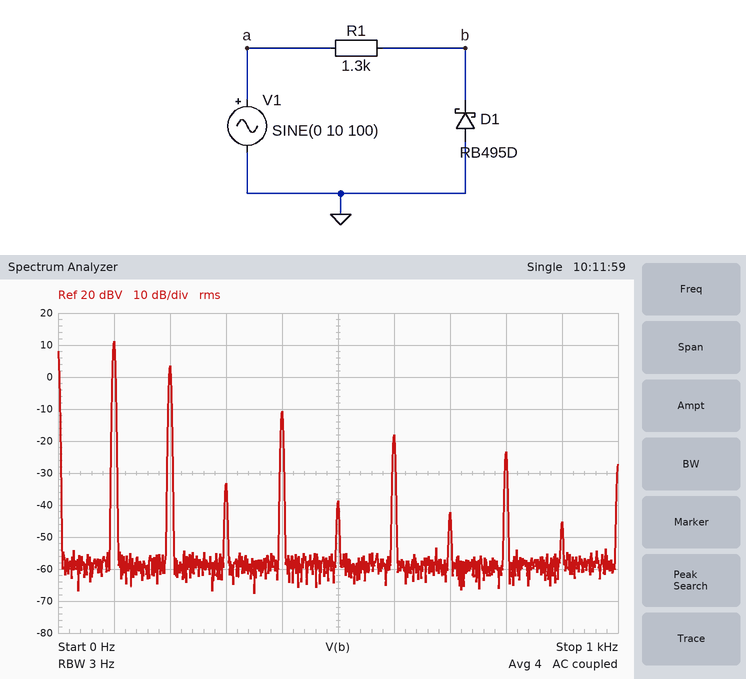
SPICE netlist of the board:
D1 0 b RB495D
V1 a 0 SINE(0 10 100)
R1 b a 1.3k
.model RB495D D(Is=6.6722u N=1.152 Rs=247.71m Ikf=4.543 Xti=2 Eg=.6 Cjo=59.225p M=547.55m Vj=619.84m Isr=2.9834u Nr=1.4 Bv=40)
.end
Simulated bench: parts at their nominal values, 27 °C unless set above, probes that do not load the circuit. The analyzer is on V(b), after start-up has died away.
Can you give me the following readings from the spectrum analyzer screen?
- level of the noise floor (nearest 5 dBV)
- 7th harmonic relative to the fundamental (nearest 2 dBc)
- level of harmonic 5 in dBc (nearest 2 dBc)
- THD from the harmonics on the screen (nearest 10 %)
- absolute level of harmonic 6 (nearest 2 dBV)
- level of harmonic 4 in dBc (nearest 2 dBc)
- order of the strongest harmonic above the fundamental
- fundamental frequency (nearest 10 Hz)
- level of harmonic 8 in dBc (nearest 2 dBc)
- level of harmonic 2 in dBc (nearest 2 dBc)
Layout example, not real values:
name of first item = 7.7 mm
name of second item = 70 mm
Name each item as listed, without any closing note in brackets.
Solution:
level of the noise floor = -60 dBV
7th harmonic relative to the fundamental = -54 dBc
level of harmonic 5 in dBc = -50 dBc
THD from the harmonics on the screen = 40 %
absolute level of harmonic 6 = -18 dBV
level of harmonic 4 in dBc = -22 dBc
order of the strongest harmonic above the fundamental = 2
fundamental frequency = 100 Hz
level of harmonic 8 in dBc = -34 dBc
level of harmonic 2 in dBc = -8 dBc
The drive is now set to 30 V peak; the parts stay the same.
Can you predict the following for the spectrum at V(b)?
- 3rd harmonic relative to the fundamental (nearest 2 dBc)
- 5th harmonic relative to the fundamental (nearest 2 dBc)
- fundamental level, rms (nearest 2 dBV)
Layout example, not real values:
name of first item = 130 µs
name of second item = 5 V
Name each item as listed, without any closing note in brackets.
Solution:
3rd harmonic relative to the fundamental = -52 dBc
5th harmonic relative to the fundamental = -58 dBc
fundamental level, rms = 20 dBV
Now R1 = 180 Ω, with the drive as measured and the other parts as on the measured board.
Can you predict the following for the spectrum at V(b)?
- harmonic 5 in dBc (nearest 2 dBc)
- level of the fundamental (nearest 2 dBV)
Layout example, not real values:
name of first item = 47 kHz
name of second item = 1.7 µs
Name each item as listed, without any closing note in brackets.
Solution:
harmonic 5 in dBc = -46 dBc
level of the fundamental = 12 dBV
